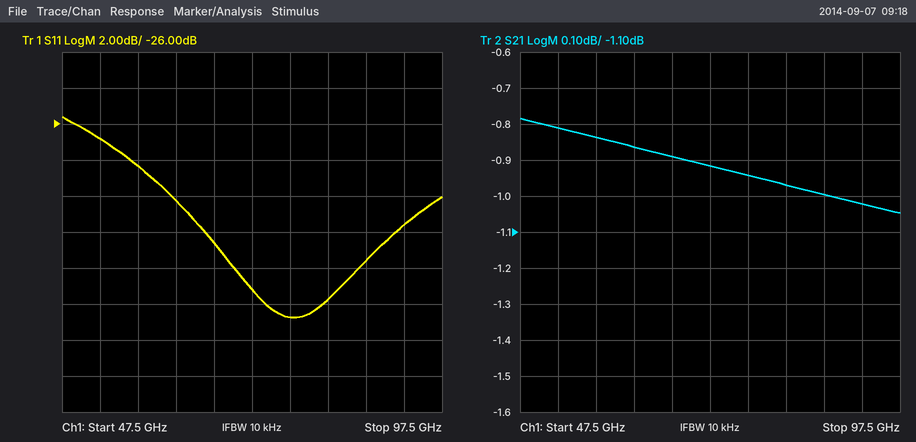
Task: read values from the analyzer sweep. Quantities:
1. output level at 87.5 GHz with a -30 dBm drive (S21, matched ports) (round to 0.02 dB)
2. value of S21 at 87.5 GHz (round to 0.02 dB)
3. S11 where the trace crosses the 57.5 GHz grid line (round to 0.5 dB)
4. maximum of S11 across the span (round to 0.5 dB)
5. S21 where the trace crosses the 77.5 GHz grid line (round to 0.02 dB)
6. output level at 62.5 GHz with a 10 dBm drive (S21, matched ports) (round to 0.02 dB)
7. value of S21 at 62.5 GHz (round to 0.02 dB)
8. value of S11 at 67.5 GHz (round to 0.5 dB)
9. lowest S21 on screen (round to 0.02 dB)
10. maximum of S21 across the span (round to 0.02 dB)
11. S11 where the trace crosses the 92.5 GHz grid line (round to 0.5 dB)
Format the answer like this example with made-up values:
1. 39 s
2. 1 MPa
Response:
1. -31.00 dBm
2. -1.00 dB
3. -28.5 dB
4. -25.5 dB
5. -0.94 dB
6. 9.14 dBm
7. -0.86 dB
8. -32.5 dB
9. -1.04 dB
10. -0.78 dB
11. -31.5 dB
